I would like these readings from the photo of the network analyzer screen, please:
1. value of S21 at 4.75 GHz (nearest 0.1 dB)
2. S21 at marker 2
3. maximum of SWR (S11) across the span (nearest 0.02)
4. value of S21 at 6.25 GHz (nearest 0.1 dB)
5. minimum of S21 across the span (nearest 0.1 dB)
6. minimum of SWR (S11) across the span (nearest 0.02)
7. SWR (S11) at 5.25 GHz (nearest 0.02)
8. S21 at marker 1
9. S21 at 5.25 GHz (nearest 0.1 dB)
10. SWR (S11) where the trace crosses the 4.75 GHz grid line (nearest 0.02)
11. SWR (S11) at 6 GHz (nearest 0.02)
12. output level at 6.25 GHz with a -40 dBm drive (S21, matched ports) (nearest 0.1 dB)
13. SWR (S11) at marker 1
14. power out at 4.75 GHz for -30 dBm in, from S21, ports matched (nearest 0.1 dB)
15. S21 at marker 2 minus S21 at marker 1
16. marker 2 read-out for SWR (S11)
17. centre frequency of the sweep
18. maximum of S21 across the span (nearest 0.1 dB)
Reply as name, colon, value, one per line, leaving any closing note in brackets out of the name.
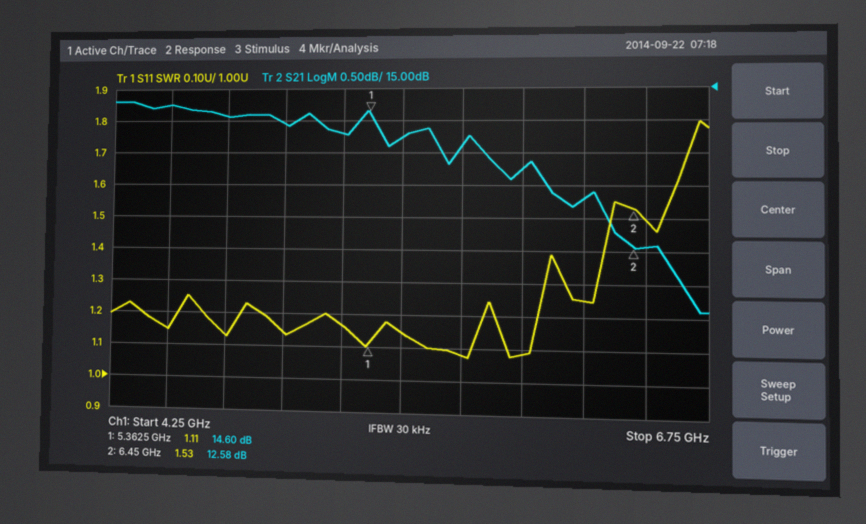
value of S21 at 4.75 GHz: 14.6 dB
S21 at marker 2: 12.58 dB
maximum of SWR (S11) across the span: 1.80
value of S21 at 6.25 GHz: 13.3 dB
minimum of S21 across the span: 11.6 dB
minimum of SWR (S11) across the span: 1.08
SWR (S11) at 5.25 GHz: 1.16
S21 at marker 1: 14.60 dB
S21 at 5.25 GHz: 14.3 dB
SWR (S11) where the trace crosses the 4.75 GHz grid line: 1.14
SWR (S11) at 6 GHz: 1.08
output level at 6.25 GHz with a -40 dBm drive (S21, matched ports): -26.7 dBm
SWR (S11) at marker 1: 1.11
power out at 4.75 GHz for -30 dBm in, from S21, ports matched: -15.4 dBm
S21 at marker 2 minus S21 at marker 1: -2.02 dB
marker 2 read-out for SWR: 1.53
centre frequency of the sweep: 5.5 GHz
maximum of S21 across the span: 14.8 dB
